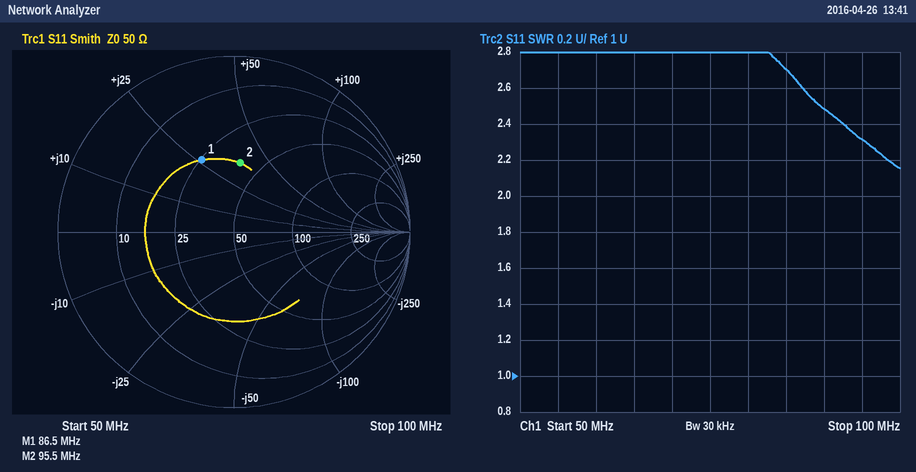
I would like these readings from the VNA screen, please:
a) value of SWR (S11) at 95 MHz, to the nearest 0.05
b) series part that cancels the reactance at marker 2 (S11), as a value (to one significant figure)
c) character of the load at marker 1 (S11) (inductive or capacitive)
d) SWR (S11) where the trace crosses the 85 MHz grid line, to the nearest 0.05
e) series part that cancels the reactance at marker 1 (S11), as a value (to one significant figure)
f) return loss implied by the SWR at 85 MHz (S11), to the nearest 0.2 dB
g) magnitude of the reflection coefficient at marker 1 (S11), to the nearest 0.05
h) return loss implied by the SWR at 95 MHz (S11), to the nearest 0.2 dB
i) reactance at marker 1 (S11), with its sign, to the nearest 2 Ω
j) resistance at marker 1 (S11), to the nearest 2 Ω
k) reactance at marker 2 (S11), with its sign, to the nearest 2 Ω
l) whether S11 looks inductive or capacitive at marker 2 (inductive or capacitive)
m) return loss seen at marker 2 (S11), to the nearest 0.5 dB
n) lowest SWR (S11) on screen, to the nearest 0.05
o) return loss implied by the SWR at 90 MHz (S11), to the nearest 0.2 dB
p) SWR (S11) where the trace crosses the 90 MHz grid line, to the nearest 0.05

2.30
50 pF
inductive
2.70
70 pF
6.8 dB
0.45
8.0 dB
+26 Ω
26 Ω
+36 Ω
inductive
8.0 dB
2.15
7.4 dB
2.50
